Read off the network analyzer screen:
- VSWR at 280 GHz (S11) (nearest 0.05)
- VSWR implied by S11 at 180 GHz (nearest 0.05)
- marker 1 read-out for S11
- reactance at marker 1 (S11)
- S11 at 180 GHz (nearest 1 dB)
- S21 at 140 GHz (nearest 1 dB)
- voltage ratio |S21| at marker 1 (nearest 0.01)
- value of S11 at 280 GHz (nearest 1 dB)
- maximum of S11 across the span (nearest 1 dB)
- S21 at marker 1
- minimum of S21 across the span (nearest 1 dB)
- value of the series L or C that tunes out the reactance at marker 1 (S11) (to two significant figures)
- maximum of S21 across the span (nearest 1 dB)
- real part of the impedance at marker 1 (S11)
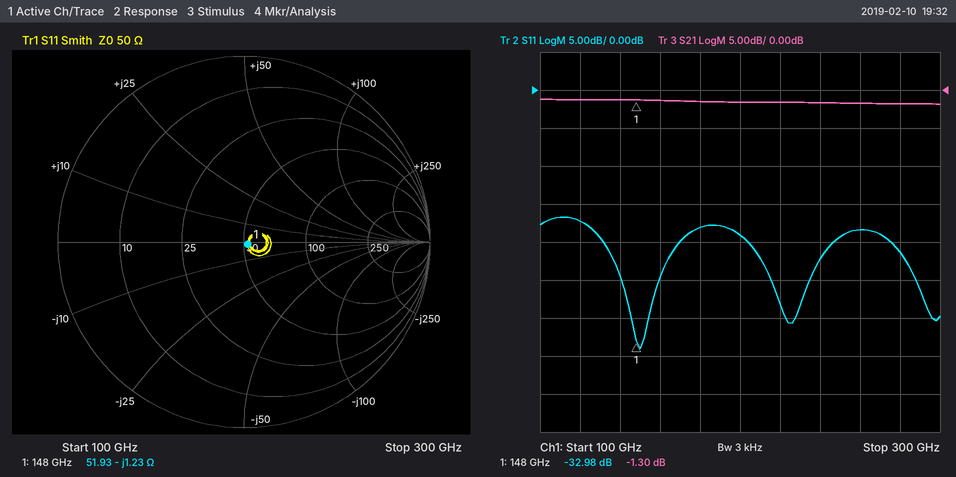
1.20
1.30
-32.98 dB
-1.23 Ω
-18 dB
-1 dB
0.86
-21 dB
-17 dB
-1.30 dB
-2 dB
1.3 pH
-1 dB
51.93 Ω
